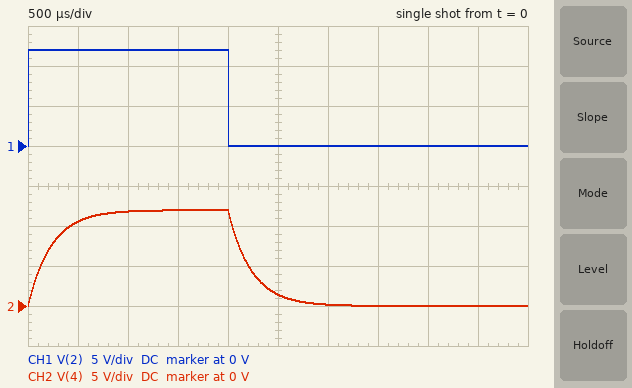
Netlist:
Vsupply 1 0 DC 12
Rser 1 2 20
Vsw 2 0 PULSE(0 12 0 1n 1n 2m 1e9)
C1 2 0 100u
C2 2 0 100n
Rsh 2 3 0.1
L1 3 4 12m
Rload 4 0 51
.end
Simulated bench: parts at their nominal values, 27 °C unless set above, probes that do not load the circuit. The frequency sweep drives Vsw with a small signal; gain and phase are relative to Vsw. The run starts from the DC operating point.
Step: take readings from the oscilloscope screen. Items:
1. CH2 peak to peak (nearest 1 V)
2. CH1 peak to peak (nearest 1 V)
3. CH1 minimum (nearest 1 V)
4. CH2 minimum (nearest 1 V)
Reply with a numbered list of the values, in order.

1. 12 V
2. 12 V
3. 0 V
4. 0 V
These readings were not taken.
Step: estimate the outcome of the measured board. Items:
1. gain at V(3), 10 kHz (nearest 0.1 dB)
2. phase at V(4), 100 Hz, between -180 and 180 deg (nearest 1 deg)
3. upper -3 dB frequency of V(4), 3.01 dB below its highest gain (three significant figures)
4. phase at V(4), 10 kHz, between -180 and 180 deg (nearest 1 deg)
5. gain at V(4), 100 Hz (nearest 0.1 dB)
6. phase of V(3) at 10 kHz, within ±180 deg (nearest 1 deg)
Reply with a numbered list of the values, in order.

1. 0 dB
2. -8 deg
3. 678 Hz
4. -86 deg
5. -0.1 dB
6. 0 deg
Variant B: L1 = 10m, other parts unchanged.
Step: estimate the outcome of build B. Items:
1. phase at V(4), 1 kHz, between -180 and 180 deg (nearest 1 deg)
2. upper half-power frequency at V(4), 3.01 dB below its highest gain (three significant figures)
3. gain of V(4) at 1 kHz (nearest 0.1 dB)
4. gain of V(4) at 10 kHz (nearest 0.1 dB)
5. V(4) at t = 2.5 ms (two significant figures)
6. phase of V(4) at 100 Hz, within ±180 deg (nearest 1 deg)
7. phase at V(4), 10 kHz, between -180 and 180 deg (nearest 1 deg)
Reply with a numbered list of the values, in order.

1. -51 deg
2. 813 Hz
3. -4.0 dB
4. -21.8 dB
5. 930 mV
6. -7 deg
7. -85 deg
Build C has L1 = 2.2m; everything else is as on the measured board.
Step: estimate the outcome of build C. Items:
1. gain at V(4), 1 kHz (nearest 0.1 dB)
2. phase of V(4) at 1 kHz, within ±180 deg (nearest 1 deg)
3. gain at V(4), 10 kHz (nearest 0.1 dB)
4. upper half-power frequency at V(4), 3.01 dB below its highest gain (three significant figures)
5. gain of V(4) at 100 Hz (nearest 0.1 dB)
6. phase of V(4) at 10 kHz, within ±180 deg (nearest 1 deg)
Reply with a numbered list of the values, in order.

1. -0.3 dB
2. -15 deg
3. -9.2 dB
4. 3.70 kHz
5. 0 dB
6. -70 deg
